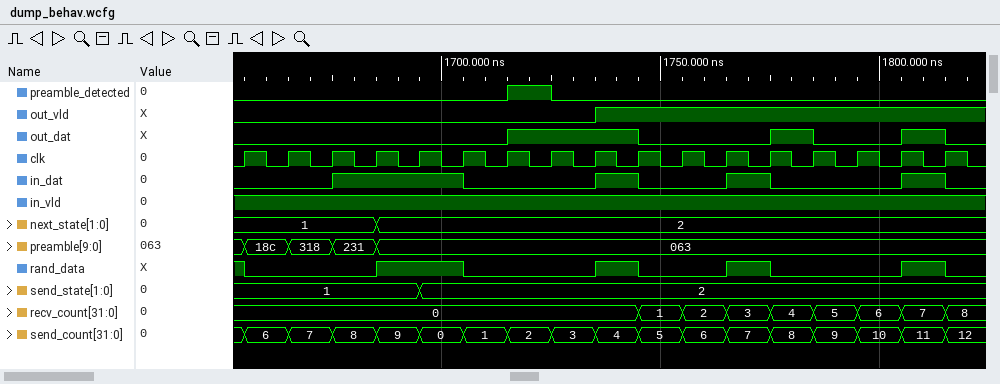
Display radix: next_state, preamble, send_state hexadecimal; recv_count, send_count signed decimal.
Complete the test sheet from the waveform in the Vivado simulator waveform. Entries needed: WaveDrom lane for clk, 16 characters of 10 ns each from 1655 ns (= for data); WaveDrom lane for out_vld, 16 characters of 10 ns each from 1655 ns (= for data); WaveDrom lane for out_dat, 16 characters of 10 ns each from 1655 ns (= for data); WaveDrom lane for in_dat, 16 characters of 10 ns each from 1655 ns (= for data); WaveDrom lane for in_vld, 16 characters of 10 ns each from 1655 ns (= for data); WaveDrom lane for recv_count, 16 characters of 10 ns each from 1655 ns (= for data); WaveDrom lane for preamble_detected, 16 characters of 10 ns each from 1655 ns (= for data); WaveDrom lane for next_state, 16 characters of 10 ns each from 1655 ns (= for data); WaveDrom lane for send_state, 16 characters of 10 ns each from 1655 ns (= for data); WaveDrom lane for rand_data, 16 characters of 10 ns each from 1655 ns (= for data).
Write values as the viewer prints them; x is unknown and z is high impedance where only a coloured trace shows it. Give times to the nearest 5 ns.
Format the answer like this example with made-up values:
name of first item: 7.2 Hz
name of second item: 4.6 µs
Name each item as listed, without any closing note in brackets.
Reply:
WaveDrom lane for clk, 16 characters of 10 ns each from 1655 ns: {name: 'clk', wave: 'p...............'}
WaveDrom lane for out_vld, 16 characters of 10 ns each from 1655 ns: {name: 'out_vld', wave: '0.......1.......'}
WaveDrom lane for out_dat, 16 characters of 10 ns each from 1655 ns: {name: 'out_dat', wave: '0.....1..0..10.1'}
WaveDrom lane for in_dat, 16 characters of 10 ns each from 1655 ns: {name: 'in_dat', wave: '0.1..0..10.10..1'}
WaveDrom lane for in_vld, 16 characters of 10 ns each from 1655 ns: {name: 'in_vld', wave: '1...............'}
WaveDrom lane for recv_count, 16 characters of 10 ns each from 1655 ns: {name: 'recv_count', wave: '=........=======', data: '0 1 2 3 4 5 6 7'}
WaveDrom lane for preamble_detected, 16 characters of 10 ns each from 1655 ns: {name: 'preamble_detected', wave: '0.....10........'}
WaveDrom lane for next_state, 16 characters of 10 ns each from 1655 ns: {name: 'next_state', wave: '=..=............', data: '1 2'}
WaveDrom lane for send_state, 16 characters of 10 ns each from 1655 ns: {name: 'send_state', wave: '=...=...........', data: '1 2'}
WaveDrom lane for rand_data, 16 characters of 10 ns each from 1655 ns: {name: 'rand_data', wave: '0..1.0..10.10..1'}
